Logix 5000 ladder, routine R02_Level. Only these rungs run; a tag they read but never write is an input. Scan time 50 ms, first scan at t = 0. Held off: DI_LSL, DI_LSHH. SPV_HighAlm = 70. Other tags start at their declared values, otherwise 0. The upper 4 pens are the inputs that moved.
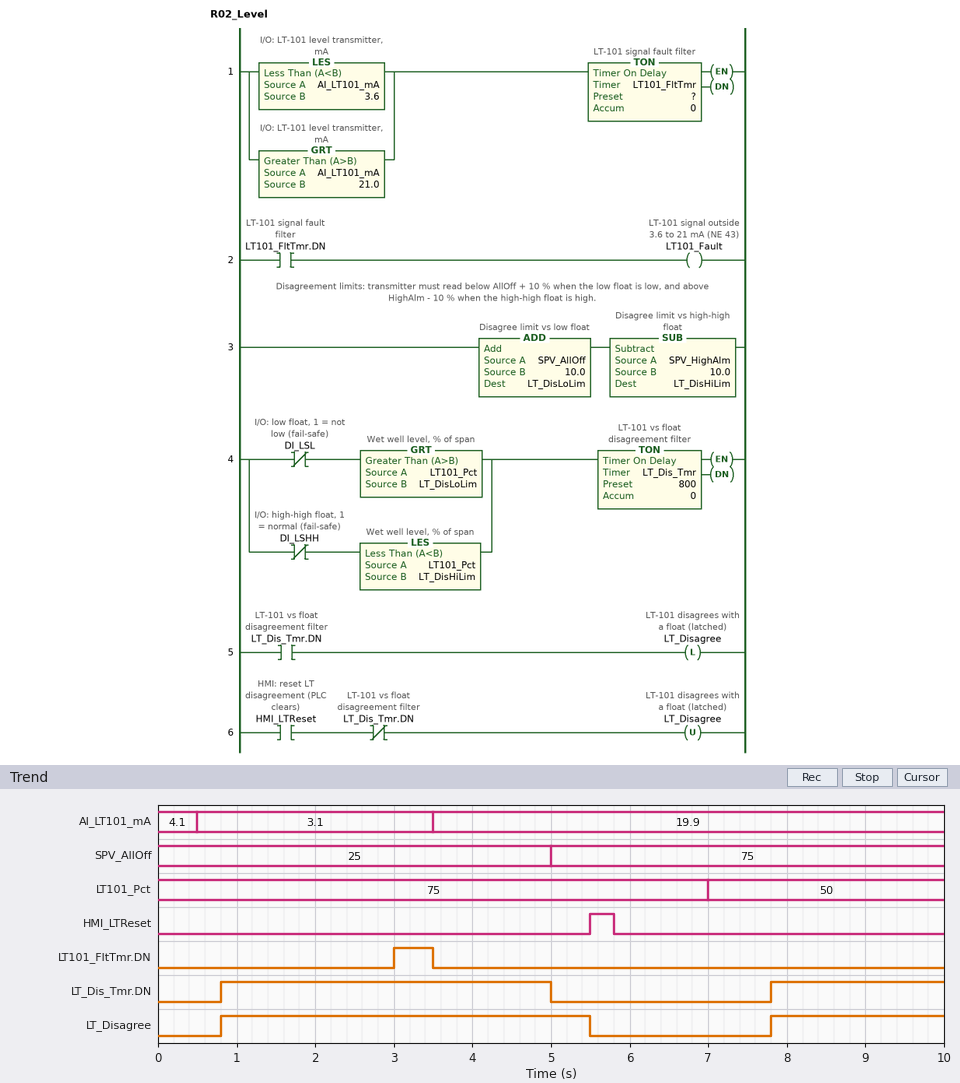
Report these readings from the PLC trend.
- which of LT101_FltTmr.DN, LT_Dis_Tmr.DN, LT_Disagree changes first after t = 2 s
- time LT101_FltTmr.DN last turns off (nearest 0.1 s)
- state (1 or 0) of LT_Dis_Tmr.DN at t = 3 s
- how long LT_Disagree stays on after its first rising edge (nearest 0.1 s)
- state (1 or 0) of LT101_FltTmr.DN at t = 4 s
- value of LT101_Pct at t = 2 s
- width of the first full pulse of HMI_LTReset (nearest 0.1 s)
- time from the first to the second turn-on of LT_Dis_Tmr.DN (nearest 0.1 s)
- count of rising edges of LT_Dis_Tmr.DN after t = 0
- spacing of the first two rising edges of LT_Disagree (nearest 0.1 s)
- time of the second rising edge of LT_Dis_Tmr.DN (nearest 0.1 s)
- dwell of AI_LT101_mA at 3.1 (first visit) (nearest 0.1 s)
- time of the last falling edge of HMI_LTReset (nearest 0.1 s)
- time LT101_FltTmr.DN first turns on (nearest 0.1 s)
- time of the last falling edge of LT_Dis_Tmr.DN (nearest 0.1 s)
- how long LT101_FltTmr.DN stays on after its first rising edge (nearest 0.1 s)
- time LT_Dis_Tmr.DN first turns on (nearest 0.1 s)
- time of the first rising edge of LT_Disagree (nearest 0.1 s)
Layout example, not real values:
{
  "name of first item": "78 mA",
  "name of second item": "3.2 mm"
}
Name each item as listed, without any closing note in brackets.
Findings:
{
  "which of LT101_FltTmr.DN, LT_Dis_Tmr.DN, LT_Disagree changes first after t = 2 s": "LT101_FltTmr.DN",
  "time LT101_FltTmr.DN last turns off": "3.5 s",
  "state (1 or 0) of LT_Dis_Tmr.DN at t = 3 s": "1",
  "how long LT_Disagree stays on after its first rising edge": "4.7 s",
  "state (1 or 0) of LT101_FltTmr.DN at t = 4 s": "0",
  "value of LT101_Pct at t = 2 s": "75",
  "width of the first full pulse of HMI_LTReset": "0.3 s",
  "time from the first to the second turn-on of LT_Dis_Tmr.DN": "7.0 s",
  "count of rising edges of LT_Dis_Tmr.DN after t = 0": "2",
  "spacing of the first two rising edges of LT_Disagree": "7.0 s",
  "time of the second rising edge of LT_Dis_Tmr.DN": "7.8 s",
  "dwell of AI_LT101_mA at 3.1 (first visit)": "3.0 s",
  "time of the last falling edge of HMI_LTReset": "5.8 s",
  "time LT101_FltTmr.DN first turns on": "3.0 s",
  "time of the last falling edge of LT_Dis_Tmr.DN": "5.0 s",
  "how long LT101_FltTmr.DN stays on after its first rising edge": "0.5 s",
  "time LT_Dis_Tmr.DN first turns on": "0.8 s",
  "time of the first rising edge of LT_Disagree": "0.8 s"
}
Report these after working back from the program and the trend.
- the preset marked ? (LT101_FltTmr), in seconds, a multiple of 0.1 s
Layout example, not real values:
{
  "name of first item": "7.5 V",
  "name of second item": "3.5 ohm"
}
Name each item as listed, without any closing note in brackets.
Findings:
{
  "the preset marked ? (LT101_FltTmr), in seconds, a multiple of 0.1 s": "2.5 s"
}
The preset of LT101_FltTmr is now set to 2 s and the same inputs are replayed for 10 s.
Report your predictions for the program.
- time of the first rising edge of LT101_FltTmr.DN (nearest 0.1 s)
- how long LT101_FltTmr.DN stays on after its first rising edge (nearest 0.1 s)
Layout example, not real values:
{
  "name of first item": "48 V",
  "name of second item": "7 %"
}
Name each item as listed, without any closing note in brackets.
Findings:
{
  "time of the first rising edge of LT101_FltTmr.DN": "2.5 s",
  "how long LT101_FltTmr.DN stays on after its first rising edge": "1.0 s"
}
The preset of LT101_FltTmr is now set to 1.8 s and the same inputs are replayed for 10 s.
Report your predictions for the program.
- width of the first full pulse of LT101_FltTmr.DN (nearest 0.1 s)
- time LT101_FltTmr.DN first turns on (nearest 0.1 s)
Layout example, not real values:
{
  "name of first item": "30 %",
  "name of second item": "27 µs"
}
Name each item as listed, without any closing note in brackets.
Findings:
{
  "width of the first full pulse of LT101_FltTmr.DN": "1.2 s",
  "time LT101_FltTmr.DN first turns on": "2.3 s"
}
